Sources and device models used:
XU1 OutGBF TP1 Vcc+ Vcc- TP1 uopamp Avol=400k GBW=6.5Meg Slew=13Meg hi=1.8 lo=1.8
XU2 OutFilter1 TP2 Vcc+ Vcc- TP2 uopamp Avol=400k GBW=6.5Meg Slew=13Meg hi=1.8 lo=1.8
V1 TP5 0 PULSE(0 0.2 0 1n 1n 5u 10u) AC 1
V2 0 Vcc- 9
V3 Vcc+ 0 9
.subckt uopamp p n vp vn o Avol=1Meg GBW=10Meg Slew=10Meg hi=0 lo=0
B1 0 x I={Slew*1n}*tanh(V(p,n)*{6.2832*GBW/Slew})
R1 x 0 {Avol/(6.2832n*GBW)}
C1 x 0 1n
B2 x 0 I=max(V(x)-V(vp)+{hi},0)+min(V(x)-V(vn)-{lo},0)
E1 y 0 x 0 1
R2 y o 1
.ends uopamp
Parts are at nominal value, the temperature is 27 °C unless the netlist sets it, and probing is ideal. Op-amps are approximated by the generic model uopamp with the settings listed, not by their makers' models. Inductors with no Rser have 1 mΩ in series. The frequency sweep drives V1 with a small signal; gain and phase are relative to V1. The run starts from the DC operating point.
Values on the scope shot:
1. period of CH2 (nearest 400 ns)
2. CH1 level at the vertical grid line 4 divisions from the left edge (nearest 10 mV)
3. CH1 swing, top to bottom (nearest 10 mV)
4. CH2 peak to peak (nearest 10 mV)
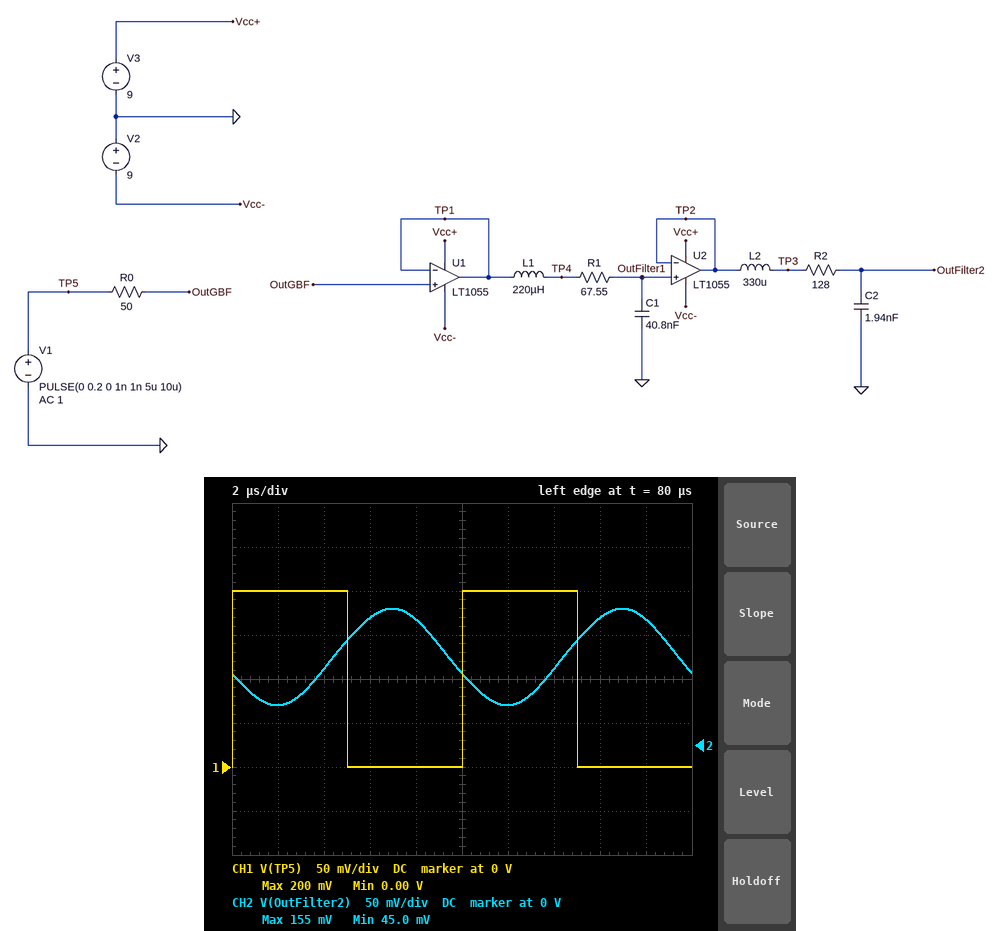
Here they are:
10.0 µs
0 V
200 mV
110 mV
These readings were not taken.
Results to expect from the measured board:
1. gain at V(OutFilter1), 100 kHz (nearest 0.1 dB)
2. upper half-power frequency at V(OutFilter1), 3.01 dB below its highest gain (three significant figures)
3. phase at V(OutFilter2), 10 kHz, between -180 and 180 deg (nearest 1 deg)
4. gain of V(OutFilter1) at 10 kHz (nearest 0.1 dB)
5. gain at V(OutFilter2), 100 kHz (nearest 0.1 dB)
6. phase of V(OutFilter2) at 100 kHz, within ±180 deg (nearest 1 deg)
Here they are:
-9.8 dB
62.7 kHz
-11 deg
0.2 dB
-7.4 dB
-159 deg
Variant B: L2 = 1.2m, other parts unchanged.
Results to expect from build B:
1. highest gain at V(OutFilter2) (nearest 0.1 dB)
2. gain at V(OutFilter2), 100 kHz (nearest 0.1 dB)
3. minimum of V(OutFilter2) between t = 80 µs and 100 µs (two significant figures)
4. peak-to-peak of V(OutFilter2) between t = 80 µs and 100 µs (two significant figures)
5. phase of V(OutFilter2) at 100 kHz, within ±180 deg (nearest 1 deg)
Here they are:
5.5 dB
5.3 dB
-140 mV
470 mV
150 deg
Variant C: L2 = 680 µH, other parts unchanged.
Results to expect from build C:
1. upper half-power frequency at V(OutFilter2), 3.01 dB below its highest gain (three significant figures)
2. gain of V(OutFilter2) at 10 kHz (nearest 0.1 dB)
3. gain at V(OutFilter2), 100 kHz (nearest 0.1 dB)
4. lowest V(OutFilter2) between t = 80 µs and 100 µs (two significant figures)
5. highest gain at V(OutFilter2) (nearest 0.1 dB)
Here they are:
69.2 kHz
0.2 dB
-3.8 dB
18 mV
2.6 dB
